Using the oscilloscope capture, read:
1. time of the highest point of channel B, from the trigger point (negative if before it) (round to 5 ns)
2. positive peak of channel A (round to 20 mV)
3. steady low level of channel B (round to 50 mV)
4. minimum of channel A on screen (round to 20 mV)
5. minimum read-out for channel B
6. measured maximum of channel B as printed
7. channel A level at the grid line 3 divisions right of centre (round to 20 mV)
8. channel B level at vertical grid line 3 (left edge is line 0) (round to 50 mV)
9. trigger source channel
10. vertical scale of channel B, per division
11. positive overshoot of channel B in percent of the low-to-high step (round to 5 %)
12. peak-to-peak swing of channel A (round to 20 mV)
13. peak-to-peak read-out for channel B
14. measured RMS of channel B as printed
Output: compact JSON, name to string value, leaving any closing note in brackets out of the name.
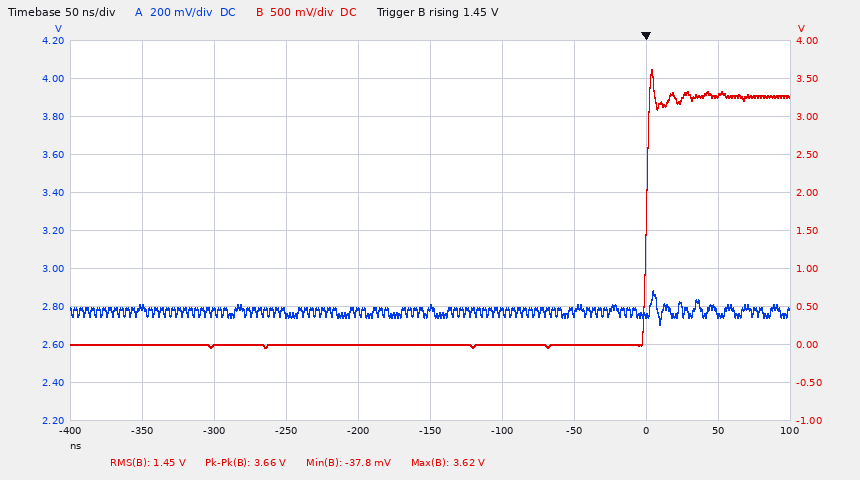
{"time of the highest point of channel B, from the trigger point (negative if before it)": "+5 ns", "positive peak of channel A": "2.88 V", "steady low level of channel B": "0 mV", "minimum of channel A on screen": "2.70 V", "minimum read-out for channel B": "-37.8 mV", "measured maximum of channel B as printed": "3.62 V", "channel A level at the grid line 3 divisions right of centre": "2.76 V", "channel B level at vertical grid line 3 (left edge is line 0)": "0 mV", "trigger source channel": "channel B", "vertical scale of channel B, per division": "500 mV", "positive overshoot of channel B in percent of the low-to-high step": "10 %", "peak-to-peak swing of channel A": "180 mV", "peak-to-peak read-out for channel B": "3.66 V", "measured RMS of channel B as printed": "1.45 V"}
